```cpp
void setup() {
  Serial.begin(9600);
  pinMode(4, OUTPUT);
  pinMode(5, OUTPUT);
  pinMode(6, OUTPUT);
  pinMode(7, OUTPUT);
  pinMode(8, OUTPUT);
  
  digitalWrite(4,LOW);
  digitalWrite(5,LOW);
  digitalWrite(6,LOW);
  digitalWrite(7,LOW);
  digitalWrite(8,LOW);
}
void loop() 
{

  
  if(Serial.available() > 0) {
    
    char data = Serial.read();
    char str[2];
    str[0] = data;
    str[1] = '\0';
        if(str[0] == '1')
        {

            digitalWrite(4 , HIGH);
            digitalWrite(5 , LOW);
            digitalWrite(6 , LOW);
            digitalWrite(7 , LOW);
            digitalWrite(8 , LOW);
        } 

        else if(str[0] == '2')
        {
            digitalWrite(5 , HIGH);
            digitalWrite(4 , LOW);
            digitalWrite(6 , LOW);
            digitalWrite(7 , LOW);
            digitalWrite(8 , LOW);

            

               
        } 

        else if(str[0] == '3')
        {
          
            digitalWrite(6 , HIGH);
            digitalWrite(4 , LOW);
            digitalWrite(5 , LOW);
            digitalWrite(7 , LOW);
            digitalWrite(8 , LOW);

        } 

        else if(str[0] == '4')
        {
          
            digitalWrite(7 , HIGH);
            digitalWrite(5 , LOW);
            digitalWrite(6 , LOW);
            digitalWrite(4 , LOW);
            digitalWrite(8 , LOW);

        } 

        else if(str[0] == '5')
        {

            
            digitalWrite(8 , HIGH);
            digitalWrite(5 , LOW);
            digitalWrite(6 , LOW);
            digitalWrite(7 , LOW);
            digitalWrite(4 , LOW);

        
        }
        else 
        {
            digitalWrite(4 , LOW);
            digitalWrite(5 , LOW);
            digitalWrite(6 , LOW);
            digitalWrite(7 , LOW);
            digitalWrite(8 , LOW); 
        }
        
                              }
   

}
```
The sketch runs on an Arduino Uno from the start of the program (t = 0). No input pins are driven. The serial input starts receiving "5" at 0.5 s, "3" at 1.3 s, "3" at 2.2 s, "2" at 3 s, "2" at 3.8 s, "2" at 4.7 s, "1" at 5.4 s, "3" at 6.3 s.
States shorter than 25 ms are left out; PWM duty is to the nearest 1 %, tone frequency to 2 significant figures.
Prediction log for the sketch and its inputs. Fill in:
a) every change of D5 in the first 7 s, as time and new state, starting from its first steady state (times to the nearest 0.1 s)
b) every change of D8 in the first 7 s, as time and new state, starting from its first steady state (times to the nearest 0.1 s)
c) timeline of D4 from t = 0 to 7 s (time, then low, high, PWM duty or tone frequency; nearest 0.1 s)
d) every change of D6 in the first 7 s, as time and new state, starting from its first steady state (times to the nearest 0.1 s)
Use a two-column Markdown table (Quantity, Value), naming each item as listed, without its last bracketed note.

| Quantity | Value |
|---|---|
| every change of D5 in the first 7 s, as time and new state, starting from its first steady state | 0 s low; 3 s high; 5.4 s low |
| every change of D8 in the first 7 s, as time and new state, starting from its first steady state | 0 s low; 0.5 s high; 1.3 s low |
| timeline of D4 from t = 0 to 7 s | 0 s low; 5.4 s high; 6.3 s low |
| every change of D6 in the first 7 s, as time and new state, starting from its first steady state | 0 s low; 1.3 s high; 3 s low; 6.3 s high |
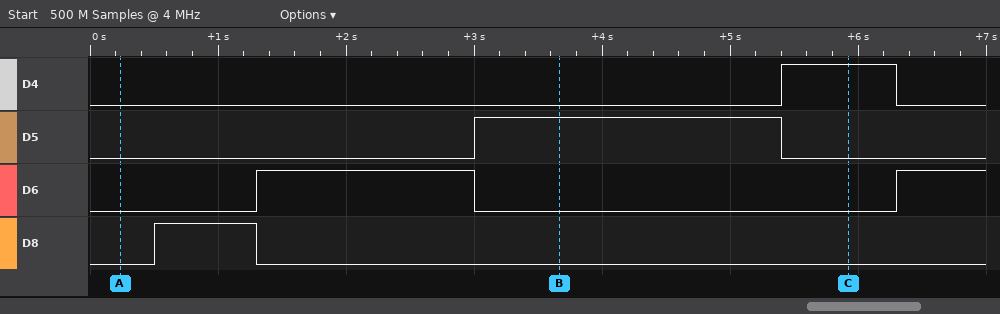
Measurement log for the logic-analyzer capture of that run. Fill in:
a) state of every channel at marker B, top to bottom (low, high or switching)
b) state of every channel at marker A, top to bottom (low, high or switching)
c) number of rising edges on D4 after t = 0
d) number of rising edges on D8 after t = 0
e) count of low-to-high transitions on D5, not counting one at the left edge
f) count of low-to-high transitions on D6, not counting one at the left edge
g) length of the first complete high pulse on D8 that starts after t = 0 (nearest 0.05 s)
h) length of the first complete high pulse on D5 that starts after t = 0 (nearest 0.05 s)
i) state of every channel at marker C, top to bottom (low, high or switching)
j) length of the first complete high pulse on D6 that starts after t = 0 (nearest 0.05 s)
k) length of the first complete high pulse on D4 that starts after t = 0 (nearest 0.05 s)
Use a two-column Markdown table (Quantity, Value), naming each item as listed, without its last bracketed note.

| Quantity | Value |
|---|---|
| state of every channel at marker B, top to bottom | D4 low, D5 high, D6 low, D8 low |
| state of every channel at marker A, top to bottom | D4 low, D5 low, D6 low, D8 low |
| number of rising edges on D4 after t = 0 | 1 |
| number of rising edges on D8 after t = 0 | 1 |
| count of low-to-high transitions on D5, not counting one at the left edge | 1 |
| count of low-to-high transitions on D6, not counting one at the left edge | 2 |
| length of the first complete high pulse on D8 that starts after t = 0 | 0.80 s |
| length of the first complete high pulse on D5 that starts after t = 0 | 2.40 s |
| state of every channel at marker C, top to bottom | D4 high, D5 low, D6 low, D8 low |
| length of the first complete high pulse on D6 that starts after t = 0 | 1.70 s |
| length of the first complete high pulse on D4 that starts after t = 0 | 0.90 s |
